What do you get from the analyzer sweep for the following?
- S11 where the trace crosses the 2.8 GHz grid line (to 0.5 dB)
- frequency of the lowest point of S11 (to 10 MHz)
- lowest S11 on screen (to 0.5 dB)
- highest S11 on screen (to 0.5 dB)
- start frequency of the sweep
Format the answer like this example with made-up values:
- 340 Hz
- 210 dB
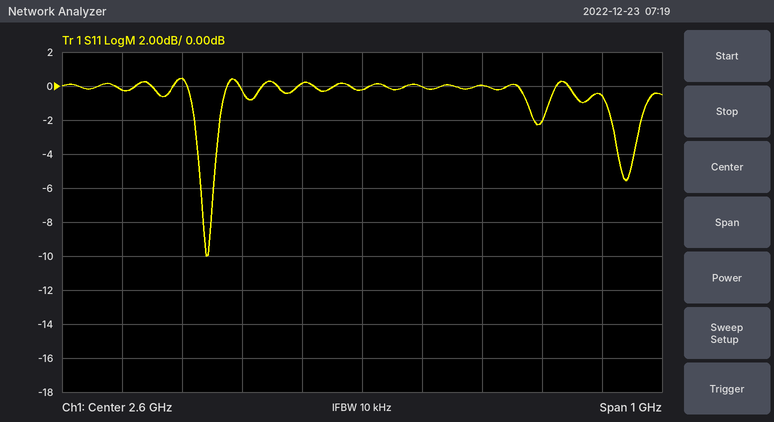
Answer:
- 0.0 dB
- 2.34 GHz
- -10.0 dB
- 0.5 dB
- 2.1 GHz
